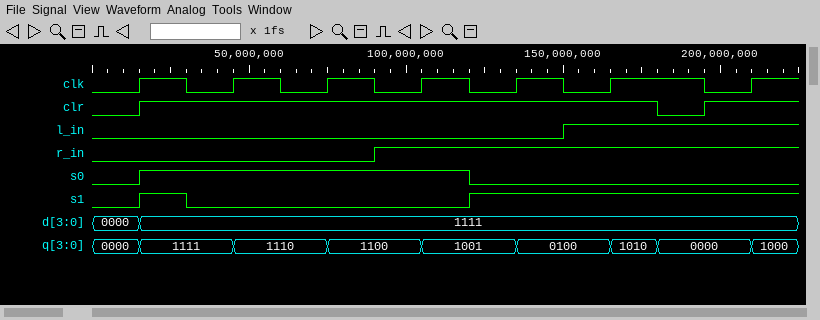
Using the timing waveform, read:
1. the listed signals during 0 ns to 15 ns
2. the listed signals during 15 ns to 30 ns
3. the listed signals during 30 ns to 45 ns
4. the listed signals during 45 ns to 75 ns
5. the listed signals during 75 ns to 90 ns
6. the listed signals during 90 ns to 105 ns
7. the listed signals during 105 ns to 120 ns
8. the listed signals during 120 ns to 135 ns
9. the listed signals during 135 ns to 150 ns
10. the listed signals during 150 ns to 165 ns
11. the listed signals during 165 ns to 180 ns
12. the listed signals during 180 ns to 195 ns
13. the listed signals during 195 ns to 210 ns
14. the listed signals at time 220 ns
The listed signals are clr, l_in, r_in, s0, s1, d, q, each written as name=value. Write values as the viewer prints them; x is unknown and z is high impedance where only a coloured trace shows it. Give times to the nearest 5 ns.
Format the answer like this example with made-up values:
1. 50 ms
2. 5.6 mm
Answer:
1. clr=0, l_in=0, r_in=0, s0=0, s1=0, d=0000, q=0000
2. clr=1, l_in=0, r_in=0, s0=1, s1=1, d=1111, q=1111
3. clr=1, l_in=0, r_in=0, s0=1, s1=0, d=1111, q=1111
4. clr=1, l_in=0, r_in=0, s0=1, s1=0, d=1111, q=1110
5. clr=1, l_in=0, r_in=0, s0=1, s1=0, d=1111, q=1100
6. clr=1, l_in=0, r_in=1, s0=1, s1=0, d=1111, q=1100
7. clr=1, l_in=0, r_in=1, s0=1, s1=0, d=1111, q=1001
8. clr=1, l_in=0, r_in=1, s0=0, s1=1, d=1111, q=1001
9. clr=1, l_in=0, r_in=1, s0=0, s1=1, d=1111, q=0100
10. clr=1, l_in=1, r_in=1, s0=0, s1=1, d=1111, q=0100
11. clr=1, l_in=1, r_in=1, s0=0, s1=1, d=1111, q=1010
12. clr=0, l_in=1, r_in=1, s0=0, s1=1, d=1111, q=0000
13. clr=1, l_in=1, r_in=1, s0=0, s1=1, d=1111, q=0000
14. clr=1, l_in=1, r_in=1, s0=0, s1=1, d=1111, q=1000
